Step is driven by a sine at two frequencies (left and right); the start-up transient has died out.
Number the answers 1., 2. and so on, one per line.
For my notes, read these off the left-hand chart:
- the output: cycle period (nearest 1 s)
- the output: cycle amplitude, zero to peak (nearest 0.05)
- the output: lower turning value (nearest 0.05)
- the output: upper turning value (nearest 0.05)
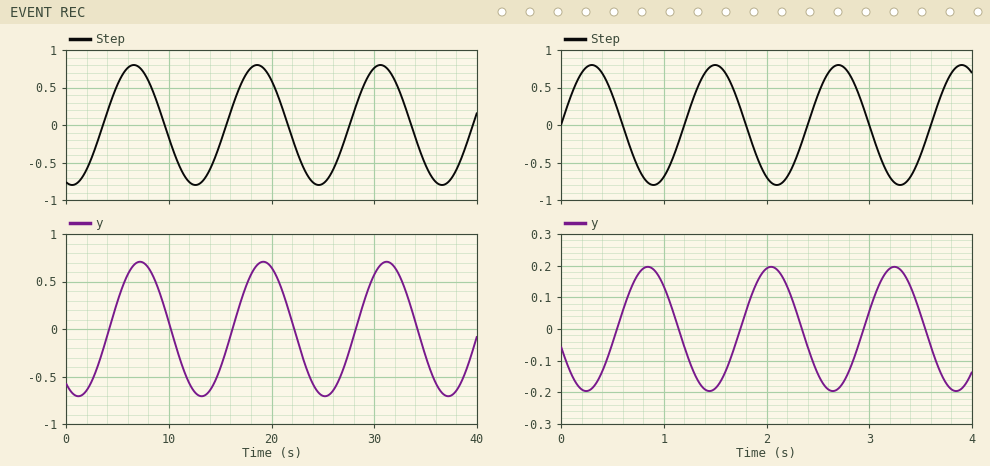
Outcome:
1. 12 s
2. 0.70
3. -0.70
4. 0.70
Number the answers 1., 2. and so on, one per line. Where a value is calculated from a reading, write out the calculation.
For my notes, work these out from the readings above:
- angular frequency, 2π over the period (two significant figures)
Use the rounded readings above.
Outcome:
1. 2π / 12 = 0.52 rad/s
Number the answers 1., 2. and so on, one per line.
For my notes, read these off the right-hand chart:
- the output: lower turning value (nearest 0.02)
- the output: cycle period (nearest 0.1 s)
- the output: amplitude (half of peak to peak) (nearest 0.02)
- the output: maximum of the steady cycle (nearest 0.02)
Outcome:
1. -0.20
2. 1.2 s
3. 0.20
4. 0.20
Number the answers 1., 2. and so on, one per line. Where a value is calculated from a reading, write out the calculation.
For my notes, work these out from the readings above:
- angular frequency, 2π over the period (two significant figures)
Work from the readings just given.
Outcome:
1. 2π / 1.2 = 5.2 rad/s
